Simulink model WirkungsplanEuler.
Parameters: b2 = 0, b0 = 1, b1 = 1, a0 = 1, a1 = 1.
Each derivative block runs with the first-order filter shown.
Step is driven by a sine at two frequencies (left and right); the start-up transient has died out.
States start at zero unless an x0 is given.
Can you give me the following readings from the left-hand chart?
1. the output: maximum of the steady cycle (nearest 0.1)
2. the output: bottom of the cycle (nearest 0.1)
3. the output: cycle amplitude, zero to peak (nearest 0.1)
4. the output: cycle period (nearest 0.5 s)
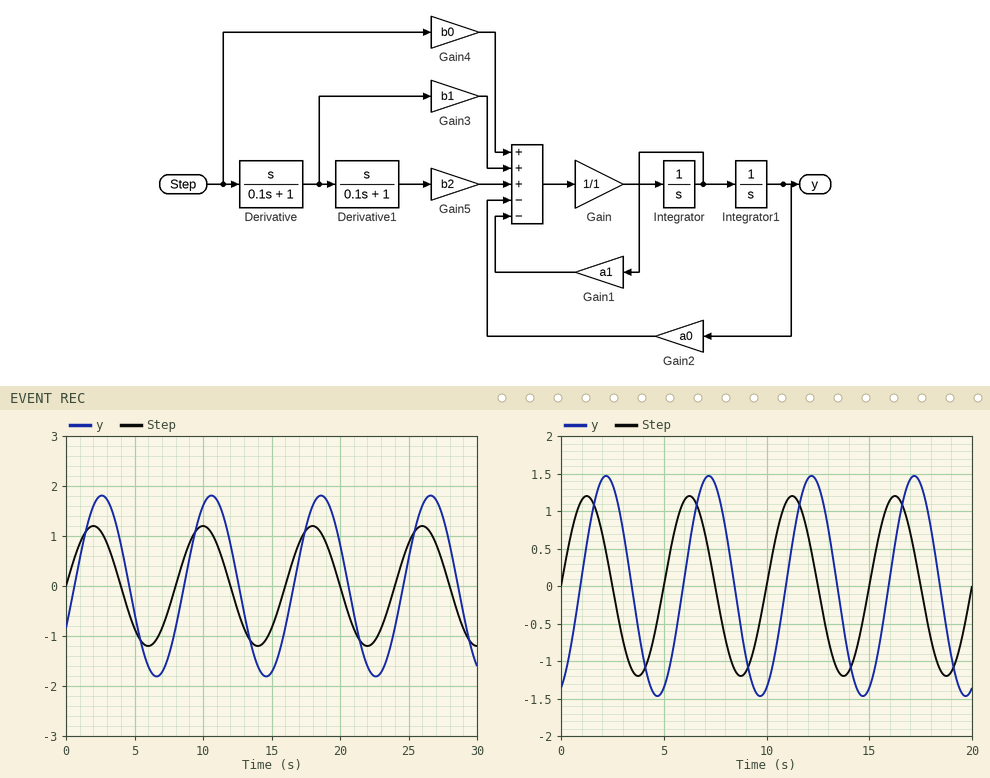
1.8
-1.8
1.8
8.0 s
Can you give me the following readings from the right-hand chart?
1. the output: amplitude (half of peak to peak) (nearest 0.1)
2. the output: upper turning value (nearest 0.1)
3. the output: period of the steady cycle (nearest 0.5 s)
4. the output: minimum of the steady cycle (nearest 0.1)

1.5
1.5
5.0 s
-1.5
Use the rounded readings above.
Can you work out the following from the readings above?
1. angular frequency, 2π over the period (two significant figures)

1.3 rad/s
